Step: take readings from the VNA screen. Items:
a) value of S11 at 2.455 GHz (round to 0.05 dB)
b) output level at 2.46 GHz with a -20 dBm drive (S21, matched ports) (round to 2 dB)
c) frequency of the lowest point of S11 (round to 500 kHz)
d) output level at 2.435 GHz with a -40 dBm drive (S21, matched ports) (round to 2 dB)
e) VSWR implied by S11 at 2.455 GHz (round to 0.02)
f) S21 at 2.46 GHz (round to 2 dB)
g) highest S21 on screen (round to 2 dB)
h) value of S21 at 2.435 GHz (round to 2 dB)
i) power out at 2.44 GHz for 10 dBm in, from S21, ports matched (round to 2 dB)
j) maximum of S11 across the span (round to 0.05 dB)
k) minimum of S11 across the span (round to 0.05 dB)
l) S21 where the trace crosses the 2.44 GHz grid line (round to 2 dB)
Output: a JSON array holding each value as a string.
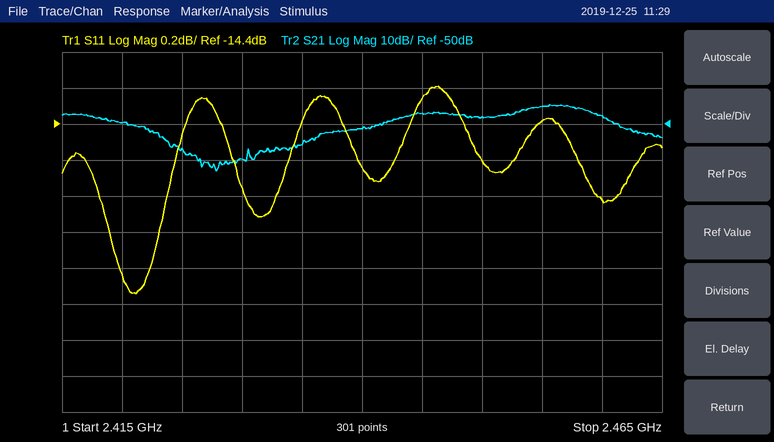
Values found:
["-14.40 dB", "-68 dBm", "2.4210 GHz", "-96 dBm", "1.48", "-48 dB", "-44 dB", "-56 dB", "-42 dBm", "-14.20 dB", "-15.35 dB", "-52 dB"]
